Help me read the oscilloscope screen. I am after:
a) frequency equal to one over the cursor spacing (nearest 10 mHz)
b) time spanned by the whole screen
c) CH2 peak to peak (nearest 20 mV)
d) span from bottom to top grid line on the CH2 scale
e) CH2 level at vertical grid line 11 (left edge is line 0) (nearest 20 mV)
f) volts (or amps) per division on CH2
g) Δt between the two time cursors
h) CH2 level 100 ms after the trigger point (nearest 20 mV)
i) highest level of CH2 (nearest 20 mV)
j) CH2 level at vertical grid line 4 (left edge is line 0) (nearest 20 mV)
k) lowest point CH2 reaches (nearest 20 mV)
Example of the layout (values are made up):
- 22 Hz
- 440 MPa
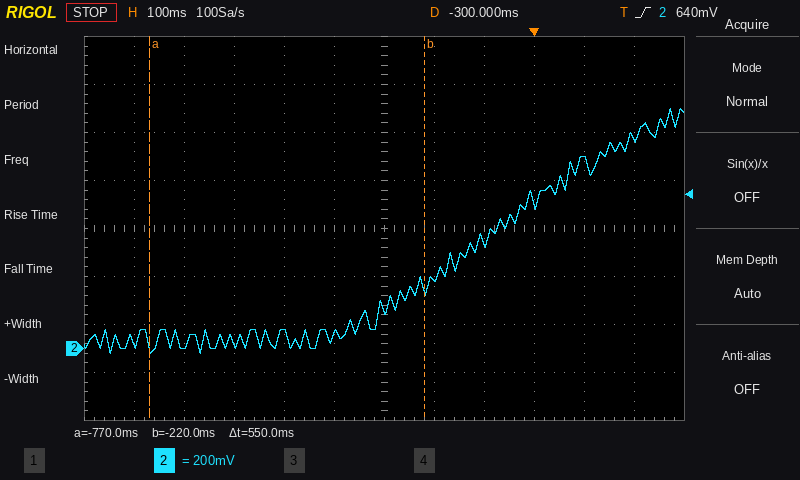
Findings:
- 1.82 Hz
- 1.2 s
- 1.02 V
- 1.6 V
- 880 mV
- 200 mV
- 550 ms
- 780 mV
- 1.00 V
- 60 mV
- -20 mV
